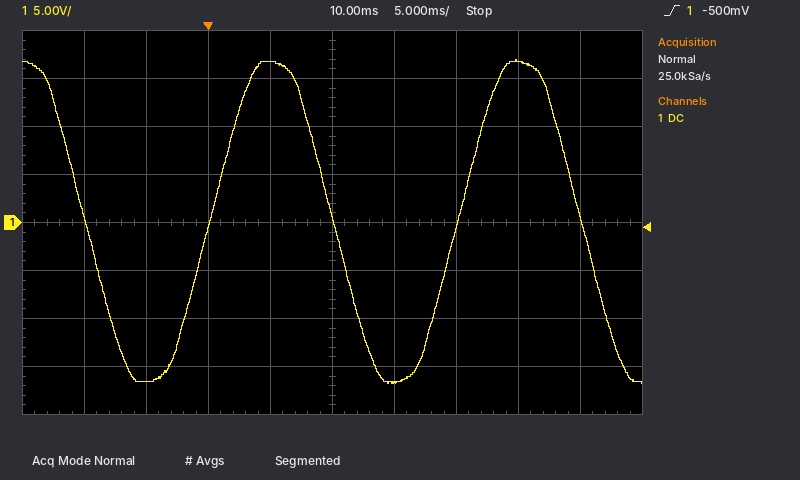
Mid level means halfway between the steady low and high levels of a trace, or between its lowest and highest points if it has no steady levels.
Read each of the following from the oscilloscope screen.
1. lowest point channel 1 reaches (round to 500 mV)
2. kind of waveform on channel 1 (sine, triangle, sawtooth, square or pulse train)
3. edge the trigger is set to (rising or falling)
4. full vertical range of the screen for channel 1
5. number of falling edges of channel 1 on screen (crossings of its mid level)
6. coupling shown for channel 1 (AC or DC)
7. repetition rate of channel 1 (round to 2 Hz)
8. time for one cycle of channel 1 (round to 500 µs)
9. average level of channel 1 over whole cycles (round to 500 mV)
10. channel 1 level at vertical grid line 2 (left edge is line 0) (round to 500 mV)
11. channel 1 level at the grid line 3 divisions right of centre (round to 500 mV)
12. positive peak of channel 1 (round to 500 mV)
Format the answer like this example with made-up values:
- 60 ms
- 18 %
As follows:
- -17.0 V
- sine
- rising
- 40 V
- 3
- DC
- 50 Hz
- 20.0 ms
- 0.0 V
- -16.5 V
- 17.0 V
- 17.0 V
